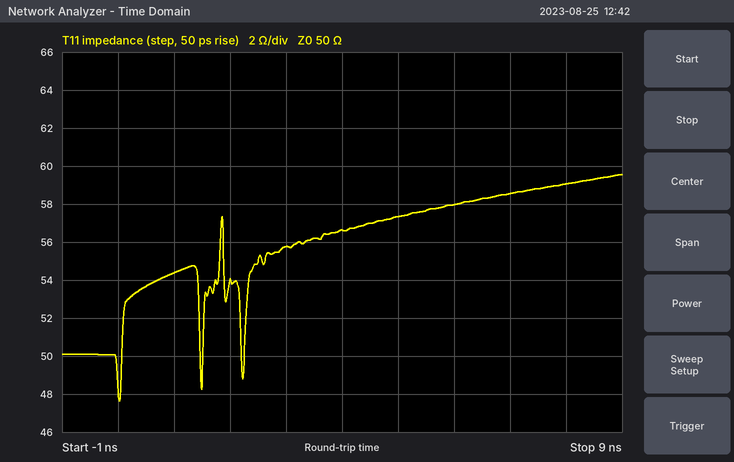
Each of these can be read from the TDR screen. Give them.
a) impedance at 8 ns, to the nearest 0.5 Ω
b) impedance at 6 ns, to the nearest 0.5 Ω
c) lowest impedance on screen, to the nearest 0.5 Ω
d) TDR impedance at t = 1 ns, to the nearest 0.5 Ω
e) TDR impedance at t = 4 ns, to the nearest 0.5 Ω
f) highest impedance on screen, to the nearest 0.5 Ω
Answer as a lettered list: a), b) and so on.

a) 59.0 Ω
b) 58.0 Ω
c) 47.5 Ω
d) 54.5 Ω
e) 56.5 Ω
f) 59.5 Ω
